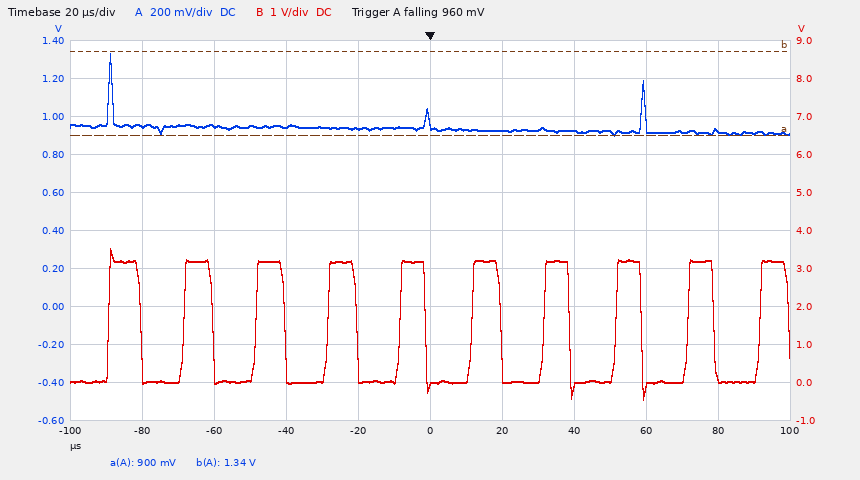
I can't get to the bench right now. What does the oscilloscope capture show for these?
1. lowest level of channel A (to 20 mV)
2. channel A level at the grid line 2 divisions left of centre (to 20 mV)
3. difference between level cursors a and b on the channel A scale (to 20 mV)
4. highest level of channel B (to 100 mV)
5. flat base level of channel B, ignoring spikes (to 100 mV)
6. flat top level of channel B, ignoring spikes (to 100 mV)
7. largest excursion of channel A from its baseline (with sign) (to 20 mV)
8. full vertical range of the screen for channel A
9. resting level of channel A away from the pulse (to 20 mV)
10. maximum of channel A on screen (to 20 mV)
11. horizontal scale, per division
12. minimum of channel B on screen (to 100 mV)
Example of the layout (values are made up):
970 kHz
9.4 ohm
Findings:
900 mV
940 mV
440 mV
3.5 V
0.0 V
3.2 V
+400 mV
2 V
940 mV
1.34 V
20 µs
-400 mV
